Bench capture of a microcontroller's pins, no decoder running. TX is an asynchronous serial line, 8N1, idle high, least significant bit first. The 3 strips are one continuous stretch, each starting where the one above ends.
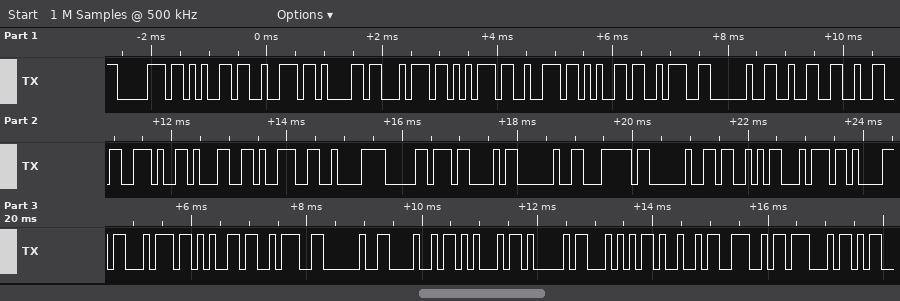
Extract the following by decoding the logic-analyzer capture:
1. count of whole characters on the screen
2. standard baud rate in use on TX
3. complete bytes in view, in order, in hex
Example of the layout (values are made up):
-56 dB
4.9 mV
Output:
35
9600 baud
70 65 72 61 74 75 72 65 3A 20 32 32 2E 31 39 C2 B0 43 20 7C 20 53 74 61 74 65 3A 20 48 45 41 54 49 4E 47
